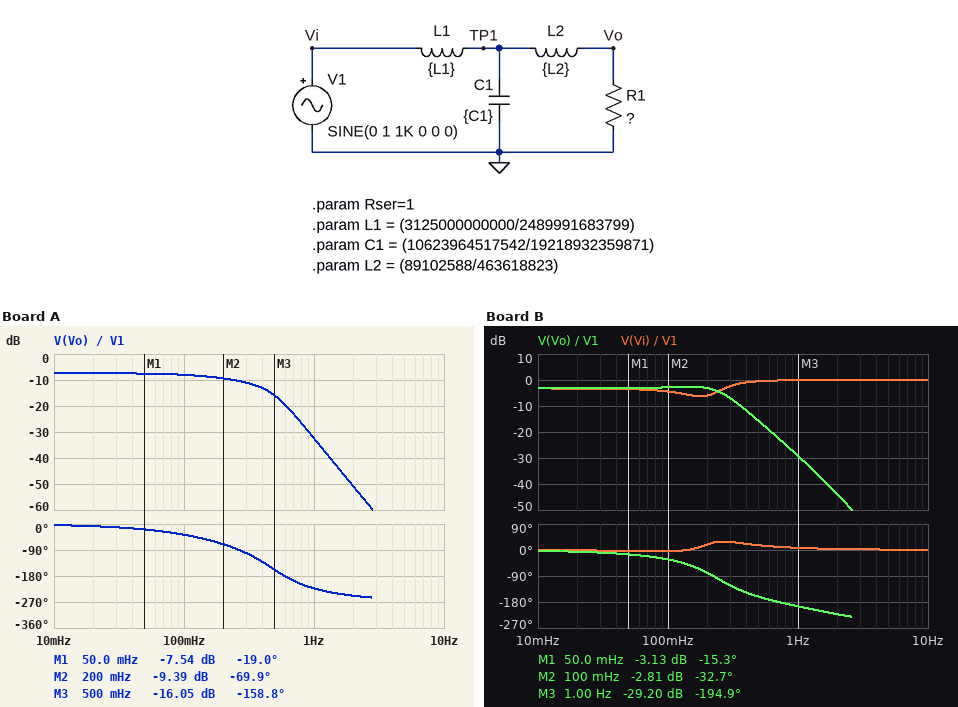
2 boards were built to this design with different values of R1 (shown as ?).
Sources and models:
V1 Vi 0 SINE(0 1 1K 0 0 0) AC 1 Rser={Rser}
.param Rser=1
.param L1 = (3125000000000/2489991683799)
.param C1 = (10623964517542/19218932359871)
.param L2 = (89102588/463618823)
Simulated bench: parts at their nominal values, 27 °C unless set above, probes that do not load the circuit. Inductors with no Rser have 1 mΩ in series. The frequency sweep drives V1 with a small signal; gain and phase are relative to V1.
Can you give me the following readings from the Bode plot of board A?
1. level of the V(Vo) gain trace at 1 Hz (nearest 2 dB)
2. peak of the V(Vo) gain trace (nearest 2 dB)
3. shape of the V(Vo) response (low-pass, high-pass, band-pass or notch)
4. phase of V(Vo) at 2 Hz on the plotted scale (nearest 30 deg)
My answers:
-32 dB
-8 dB
low-pass
-240 deg
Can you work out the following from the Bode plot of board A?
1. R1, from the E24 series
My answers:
0.75 Ω
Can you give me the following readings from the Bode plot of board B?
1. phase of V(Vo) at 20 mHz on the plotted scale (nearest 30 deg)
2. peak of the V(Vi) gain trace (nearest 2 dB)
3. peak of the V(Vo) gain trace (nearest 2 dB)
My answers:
0 deg
0 dB
-2 dB
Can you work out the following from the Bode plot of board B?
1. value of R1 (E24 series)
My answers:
2.2 Ω
